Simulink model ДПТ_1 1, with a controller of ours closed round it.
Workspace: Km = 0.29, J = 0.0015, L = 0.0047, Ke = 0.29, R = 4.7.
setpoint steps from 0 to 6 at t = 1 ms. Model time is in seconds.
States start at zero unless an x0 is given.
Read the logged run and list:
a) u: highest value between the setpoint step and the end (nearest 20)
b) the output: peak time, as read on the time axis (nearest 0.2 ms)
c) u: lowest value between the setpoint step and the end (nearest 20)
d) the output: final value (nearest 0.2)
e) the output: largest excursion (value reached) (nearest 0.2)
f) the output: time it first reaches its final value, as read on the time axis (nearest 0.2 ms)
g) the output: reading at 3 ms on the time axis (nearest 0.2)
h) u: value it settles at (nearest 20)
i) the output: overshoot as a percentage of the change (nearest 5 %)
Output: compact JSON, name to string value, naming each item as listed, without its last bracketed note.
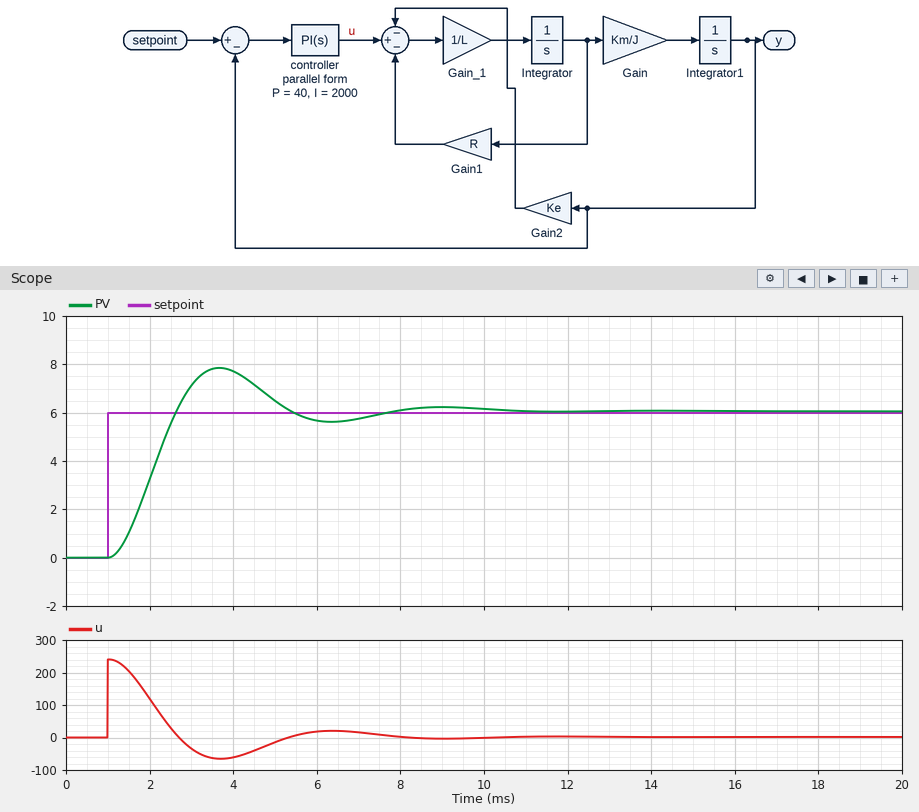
{"u: highest value between the setpoint step and the end": "240", "the output: peak time, as read on the time axis": "3.6 ms", "u: lowest value between the setpoint step and the end": "-60", "the output: final value": "6.0", "the output: largest excursion (value reached)": "7.8", "the output: time it first reaches its final value, as read on the time axis": "2.6 ms", "the output: reading at 3 ms on the time axis": "7.2", "u: value it settles at": "0", "the output: overshoot as a percentage of the change": "30 %"}
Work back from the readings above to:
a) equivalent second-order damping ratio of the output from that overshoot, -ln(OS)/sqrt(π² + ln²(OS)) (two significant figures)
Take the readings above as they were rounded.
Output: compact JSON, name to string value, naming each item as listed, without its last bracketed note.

{"equivalent second-order damping ratio of the output from that overshoot, -ln(OS)/sqrt(π² + ln²(OS))": "0.36"}
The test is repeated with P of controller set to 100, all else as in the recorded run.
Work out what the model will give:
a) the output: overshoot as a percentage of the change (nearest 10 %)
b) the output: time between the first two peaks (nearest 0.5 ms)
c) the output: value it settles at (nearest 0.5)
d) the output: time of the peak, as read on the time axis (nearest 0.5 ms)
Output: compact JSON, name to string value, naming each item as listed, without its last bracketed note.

{"the output: overshoot as a percentage of the change": "50 %", "the output: time between the first two peaks": "3.0 ms", "the output: value it settles at": "6.0", "the output: time of the peak, as read on the time axis": "2.5 ms"}
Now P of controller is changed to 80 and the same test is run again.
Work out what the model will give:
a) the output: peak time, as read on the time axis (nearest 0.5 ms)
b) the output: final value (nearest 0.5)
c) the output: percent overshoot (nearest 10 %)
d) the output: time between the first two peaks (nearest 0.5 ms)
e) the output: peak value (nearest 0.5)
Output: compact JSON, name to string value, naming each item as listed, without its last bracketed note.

{"the output: peak time, as read on the time axis": "3.0 ms", "the output: final value": "6.0", "the output: percent overshoot": "40 %", "the output: time between the first two peaks": "3.5 ms", "the output: peak value": "8.5"}
